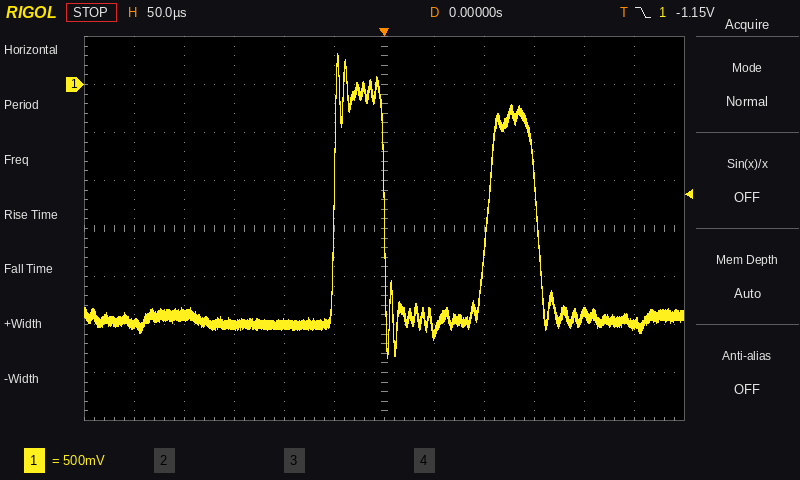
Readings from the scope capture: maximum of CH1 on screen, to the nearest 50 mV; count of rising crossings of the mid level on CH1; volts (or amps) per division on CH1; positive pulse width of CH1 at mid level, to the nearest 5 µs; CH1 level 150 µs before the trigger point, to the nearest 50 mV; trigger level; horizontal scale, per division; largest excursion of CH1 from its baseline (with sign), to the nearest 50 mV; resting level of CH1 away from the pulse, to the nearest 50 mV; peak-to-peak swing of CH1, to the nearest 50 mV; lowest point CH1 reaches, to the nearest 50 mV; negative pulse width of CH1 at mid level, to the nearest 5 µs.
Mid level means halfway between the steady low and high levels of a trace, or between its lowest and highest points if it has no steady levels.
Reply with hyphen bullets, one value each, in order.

- 300 mV
- 2
- 500 mV
- 50 µs
- -2.50 V
- -1.15 V
- 50 µs
- +2.75 V
- -2.45 V
- 3.15 V
- -2.85 V
- 105 µs
